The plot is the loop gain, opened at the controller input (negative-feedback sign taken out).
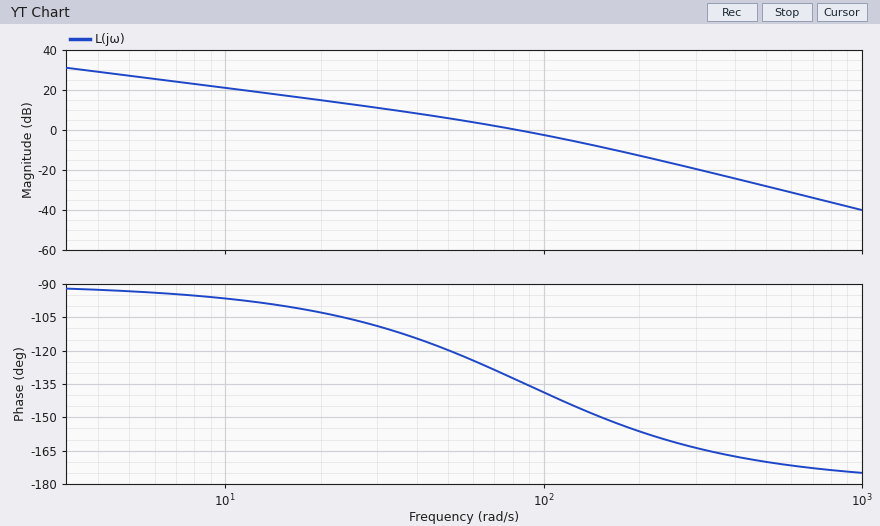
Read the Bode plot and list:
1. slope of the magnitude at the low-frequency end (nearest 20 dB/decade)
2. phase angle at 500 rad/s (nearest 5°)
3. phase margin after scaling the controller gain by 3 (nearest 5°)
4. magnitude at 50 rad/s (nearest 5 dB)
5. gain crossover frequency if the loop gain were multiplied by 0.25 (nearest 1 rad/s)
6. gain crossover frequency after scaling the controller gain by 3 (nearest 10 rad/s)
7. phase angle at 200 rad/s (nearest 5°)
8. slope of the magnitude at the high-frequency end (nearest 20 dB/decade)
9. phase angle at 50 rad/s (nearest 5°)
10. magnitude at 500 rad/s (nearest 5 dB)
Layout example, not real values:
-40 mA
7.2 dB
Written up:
-20 dB/decade
-170°
30°
5 dB
27 rad/s
160 rad/s
-155°
-40 dB/decade
-120°
-30 dB
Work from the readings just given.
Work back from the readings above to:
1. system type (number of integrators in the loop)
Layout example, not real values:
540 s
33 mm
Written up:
1
